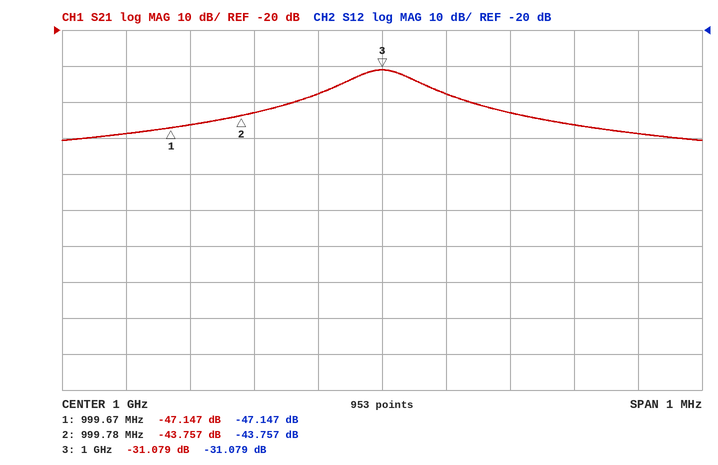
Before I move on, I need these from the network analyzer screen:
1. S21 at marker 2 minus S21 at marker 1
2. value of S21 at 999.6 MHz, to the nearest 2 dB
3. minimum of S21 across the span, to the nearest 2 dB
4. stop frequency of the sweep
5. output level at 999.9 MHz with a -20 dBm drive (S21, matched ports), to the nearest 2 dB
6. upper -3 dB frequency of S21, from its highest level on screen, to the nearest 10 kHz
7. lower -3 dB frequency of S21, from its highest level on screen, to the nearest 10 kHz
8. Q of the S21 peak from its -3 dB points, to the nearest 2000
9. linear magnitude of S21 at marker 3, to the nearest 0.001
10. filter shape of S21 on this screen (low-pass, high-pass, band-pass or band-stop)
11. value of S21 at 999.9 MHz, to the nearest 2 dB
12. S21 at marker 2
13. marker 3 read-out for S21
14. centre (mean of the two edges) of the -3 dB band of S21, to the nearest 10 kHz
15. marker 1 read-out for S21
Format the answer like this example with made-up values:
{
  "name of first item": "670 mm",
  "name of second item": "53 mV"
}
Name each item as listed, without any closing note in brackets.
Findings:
{
  "S21 at marker 2 minus S21 at marker 1": "3.390 dB",
  "value of S21 at 999.6 MHz, to the nearest 2 dB": "-48 dB",
  "minimum of S21 across the span, to the nearest 2 dB": "-50 dB",
  "stop frequency of the sweep": "1.0005 GHz",
  "output level at 999.9 MHz with a -20 dBm drive (S21, matched ports), to the nearest 2 dB": "-58 dBm",
  "upper -3 dB frequency of S21, from its highest level on screen, to the nearest 10 kHz": "1.00005 GHz",
  "lower -3 dB frequency of S21, from its highest level on screen, to the nearest 10 kHz": "999.95 MHz",
  "Q of the S21 peak from its -3 dB points, to the nearest 2000": "10000",
  "linear magnitude of S21 at marker 3, to the nearest 0.001": "0.028",
  "filter shape of S21 on this screen": "band-pass",
  "value of S21 at 999.9 MHz, to the nearest 2 dB": "-38 dB",
  "S21 at marker 2": "-43.757 dB",
  "marker 3 read-out for S21": "-31.079 dB",
  "centre (mean of the two edges) of the -3 dB band of S21, to the nearest 10 kHz": "1.00000 GHz",
  "marker 1 read-out for S21": "-47.147 dB"
}
